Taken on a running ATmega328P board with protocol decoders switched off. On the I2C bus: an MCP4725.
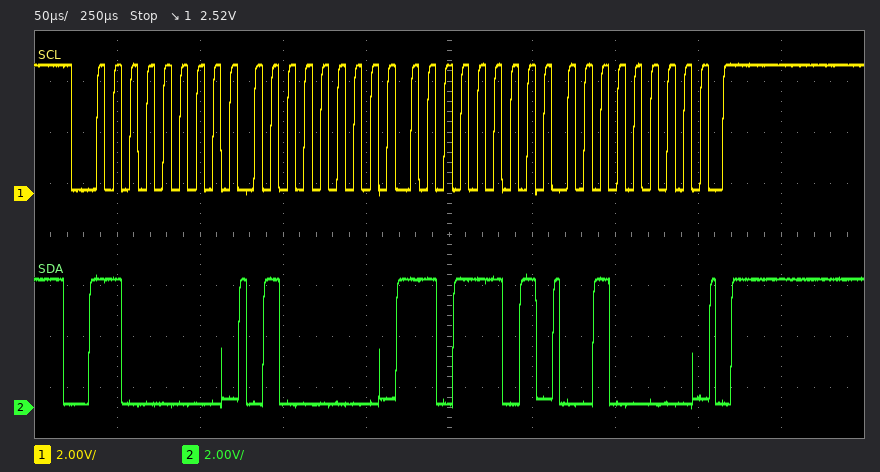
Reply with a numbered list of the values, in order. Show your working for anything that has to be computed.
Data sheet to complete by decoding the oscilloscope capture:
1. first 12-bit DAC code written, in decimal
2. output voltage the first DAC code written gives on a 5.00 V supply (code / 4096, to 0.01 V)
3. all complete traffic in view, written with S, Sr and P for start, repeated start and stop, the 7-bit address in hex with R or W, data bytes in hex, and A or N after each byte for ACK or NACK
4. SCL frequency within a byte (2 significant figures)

1. 3538
2. 3538 / 4096 x 5.00 V = 4.32 V
3. S 60W A 40 A DD A 20 A P
4. 100 kHz
